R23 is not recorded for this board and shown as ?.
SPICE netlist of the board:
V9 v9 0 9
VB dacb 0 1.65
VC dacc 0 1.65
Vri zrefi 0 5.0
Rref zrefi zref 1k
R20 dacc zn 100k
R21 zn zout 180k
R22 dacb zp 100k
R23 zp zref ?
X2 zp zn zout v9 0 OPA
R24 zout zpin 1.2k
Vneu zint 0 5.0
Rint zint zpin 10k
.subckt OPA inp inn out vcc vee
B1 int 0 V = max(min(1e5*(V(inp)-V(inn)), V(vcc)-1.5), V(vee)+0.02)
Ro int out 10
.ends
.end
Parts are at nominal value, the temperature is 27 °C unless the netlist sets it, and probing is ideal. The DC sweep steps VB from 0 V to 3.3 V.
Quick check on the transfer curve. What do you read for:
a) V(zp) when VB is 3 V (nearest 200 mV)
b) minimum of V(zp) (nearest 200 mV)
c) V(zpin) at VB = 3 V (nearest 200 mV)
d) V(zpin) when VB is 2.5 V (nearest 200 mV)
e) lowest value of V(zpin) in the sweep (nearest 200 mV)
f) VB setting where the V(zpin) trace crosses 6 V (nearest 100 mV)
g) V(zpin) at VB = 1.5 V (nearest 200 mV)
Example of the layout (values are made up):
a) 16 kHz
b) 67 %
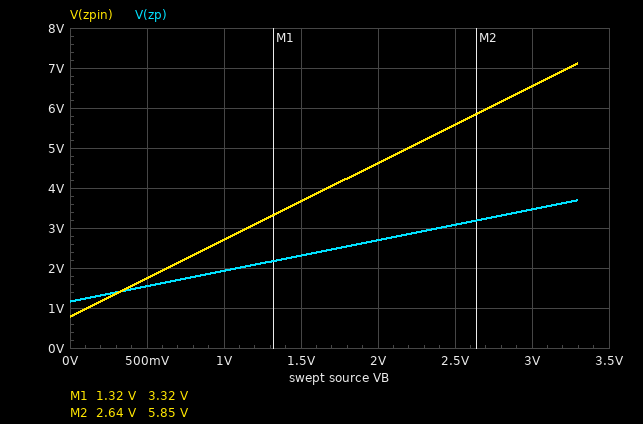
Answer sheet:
a) 3.4 V
b) 1.2 V
c) 6.6 V
d) 5.6 V
e) 800 mV
f) 2.7 V
g) 3.6 V
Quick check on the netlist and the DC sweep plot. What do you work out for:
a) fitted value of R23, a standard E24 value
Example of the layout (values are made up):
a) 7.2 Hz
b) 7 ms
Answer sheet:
a) 330 kΩ
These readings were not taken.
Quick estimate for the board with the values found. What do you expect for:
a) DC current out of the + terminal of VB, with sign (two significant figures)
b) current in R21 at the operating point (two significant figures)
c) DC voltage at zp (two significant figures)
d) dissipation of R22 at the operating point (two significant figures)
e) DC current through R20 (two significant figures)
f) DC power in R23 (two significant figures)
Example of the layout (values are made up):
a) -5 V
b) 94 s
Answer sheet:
a) -7.8 µA
b) 7.8 µA
c) 2.4 V
d) 6.0 µW
e) 7.8 µA
f) 20 µW
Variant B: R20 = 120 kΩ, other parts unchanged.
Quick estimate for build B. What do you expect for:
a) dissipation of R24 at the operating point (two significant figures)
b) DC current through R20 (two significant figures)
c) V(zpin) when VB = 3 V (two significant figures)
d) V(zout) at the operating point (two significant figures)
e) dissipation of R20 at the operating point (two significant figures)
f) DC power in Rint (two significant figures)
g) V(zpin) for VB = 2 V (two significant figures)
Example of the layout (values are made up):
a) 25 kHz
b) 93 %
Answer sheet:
a) 19 µW
b) 6.5 µA
c) 6.1 V
d) 3.6 V
e) 5.0 µW
f) 160 µW
g) 4.3 V
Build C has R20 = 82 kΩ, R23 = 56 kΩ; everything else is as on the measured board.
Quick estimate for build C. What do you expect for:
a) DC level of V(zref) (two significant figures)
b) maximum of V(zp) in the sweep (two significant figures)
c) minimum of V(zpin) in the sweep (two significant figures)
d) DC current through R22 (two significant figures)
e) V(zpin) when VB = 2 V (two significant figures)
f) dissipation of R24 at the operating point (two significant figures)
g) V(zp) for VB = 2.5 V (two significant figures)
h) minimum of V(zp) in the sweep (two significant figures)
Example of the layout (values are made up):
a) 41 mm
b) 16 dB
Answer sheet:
a) 5.0 V
b) 4.4 V
c) 6.4 V
d) 21 µA
e) 7.2 V
f) 60 µW
g) 4.1 V
h) 3.2 V
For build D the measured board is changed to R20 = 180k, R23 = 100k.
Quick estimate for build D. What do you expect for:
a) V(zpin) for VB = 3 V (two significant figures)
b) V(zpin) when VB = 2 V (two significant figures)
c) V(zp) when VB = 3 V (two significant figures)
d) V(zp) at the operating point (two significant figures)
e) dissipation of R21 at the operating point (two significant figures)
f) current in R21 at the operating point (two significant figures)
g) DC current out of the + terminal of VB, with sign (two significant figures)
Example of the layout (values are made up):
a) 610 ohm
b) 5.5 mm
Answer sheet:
a) 6.2 V
b) 5.3 V
c) 4.0 V
d) 3.3 V
e) 15 µW
f) 9.3 µA
g) -17 µA
